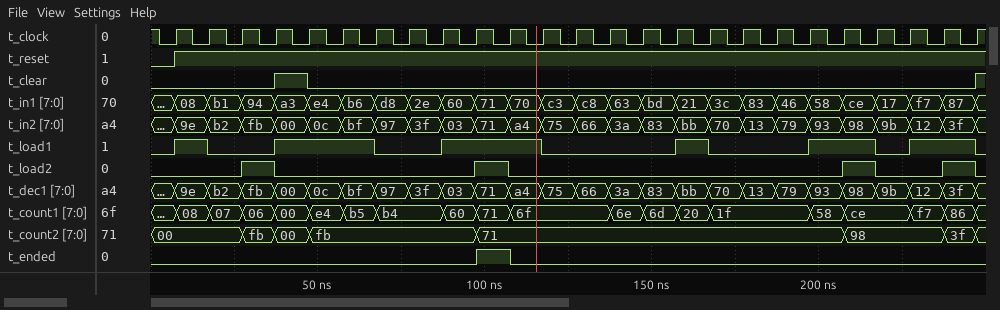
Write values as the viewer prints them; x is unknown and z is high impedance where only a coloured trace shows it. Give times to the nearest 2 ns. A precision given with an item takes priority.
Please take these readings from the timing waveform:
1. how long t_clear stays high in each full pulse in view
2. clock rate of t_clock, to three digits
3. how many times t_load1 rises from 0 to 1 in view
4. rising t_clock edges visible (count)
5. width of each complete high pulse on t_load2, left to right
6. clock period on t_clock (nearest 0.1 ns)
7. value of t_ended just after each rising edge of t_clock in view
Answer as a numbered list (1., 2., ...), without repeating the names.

1. 10 ns
2. 100 MHz
3. 6
4. 25
5. 10 ns, 10 ns, 10 ns, 10 ns
6. 10 ns
7. 0 0 0 0 0 0 0 0 0 1 0 0 0 0 0 0 0 0 0 0 0 0 0 0 0
